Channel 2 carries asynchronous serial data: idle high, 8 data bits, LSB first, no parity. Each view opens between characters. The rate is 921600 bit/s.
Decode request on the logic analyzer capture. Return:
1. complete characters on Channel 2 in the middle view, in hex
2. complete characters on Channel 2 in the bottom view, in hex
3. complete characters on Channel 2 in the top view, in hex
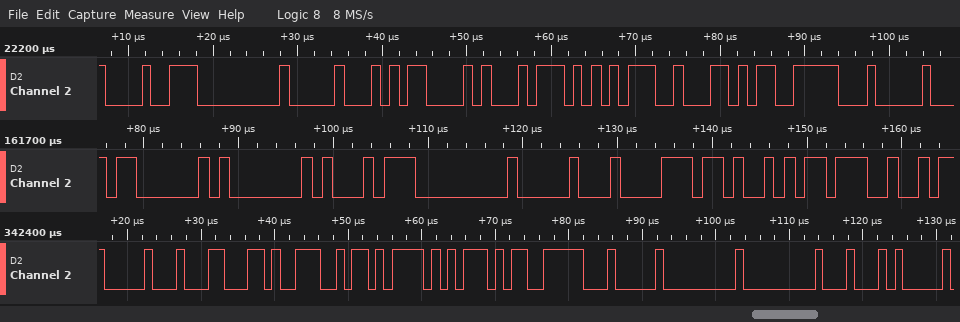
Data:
03, 01, D1, 00, 10, B8, A9, 27
10, 8C, 39, EB, 75, F3, 04, 00, 00, 44
C8, 00, 10, 0D, D1, D5, 62, F3, 04
